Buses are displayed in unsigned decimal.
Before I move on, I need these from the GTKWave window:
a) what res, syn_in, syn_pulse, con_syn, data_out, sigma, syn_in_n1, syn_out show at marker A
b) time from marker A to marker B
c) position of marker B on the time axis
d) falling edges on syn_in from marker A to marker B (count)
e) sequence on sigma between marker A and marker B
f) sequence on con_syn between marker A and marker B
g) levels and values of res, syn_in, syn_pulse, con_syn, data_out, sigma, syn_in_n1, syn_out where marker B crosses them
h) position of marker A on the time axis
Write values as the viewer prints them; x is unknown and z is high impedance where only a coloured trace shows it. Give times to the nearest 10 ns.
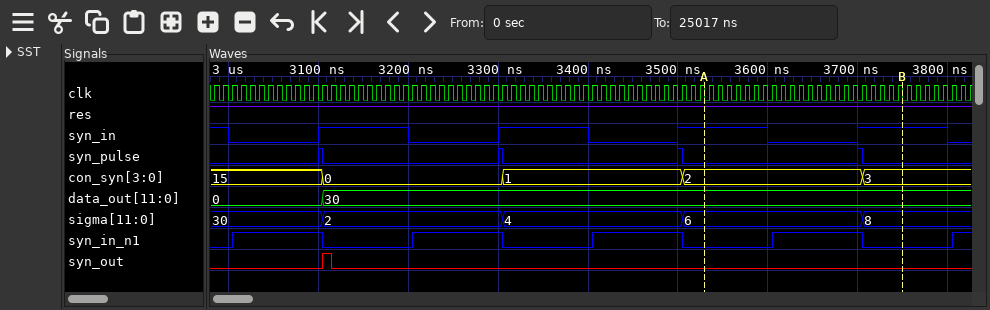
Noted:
res=1, syn_in=1, syn_pulse=0, con_syn=2, data_out=30, sigma=6, syn_in_n1=0, syn_out=0
220 ns
3750 ns
1
6, 8
2, 3
res=1, syn_in=1, syn_pulse=0, con_syn=3, data_out=30, sigma=8, syn_in_n1=0, syn_out=0
3530 ns
